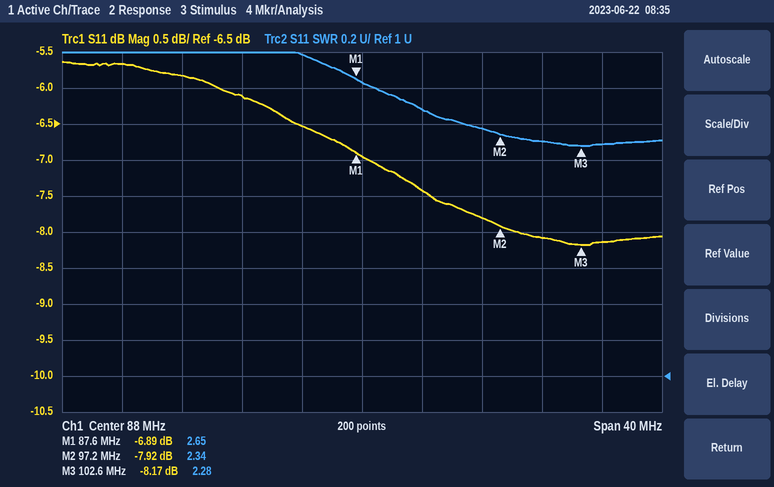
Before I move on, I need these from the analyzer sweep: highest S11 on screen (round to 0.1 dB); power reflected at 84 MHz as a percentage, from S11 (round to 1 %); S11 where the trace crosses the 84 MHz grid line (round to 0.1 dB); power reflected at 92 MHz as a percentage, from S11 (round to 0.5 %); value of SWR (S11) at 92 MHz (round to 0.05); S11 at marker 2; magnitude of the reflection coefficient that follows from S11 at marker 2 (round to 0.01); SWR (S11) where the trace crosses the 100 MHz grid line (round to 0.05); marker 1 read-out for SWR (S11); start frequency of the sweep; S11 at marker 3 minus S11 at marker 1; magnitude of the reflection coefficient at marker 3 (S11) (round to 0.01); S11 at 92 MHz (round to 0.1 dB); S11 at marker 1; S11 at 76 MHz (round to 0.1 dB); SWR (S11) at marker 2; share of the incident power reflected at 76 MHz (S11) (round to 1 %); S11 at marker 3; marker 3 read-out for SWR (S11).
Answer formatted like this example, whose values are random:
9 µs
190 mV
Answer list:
-5.6 dB
22 %
-6.5 dB
18.0 %
2.50
-7.92 dB
0.40
2.30
2.65
68 MHz
-1.28 dB
0.39
-7.4 dB
-6.89 dB
-5.8 dB
2.34
26 %
-8.17 dB
2.28
